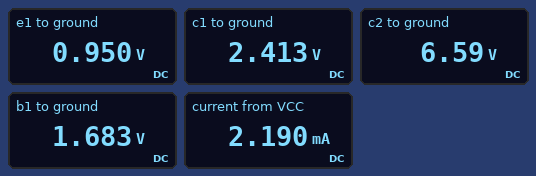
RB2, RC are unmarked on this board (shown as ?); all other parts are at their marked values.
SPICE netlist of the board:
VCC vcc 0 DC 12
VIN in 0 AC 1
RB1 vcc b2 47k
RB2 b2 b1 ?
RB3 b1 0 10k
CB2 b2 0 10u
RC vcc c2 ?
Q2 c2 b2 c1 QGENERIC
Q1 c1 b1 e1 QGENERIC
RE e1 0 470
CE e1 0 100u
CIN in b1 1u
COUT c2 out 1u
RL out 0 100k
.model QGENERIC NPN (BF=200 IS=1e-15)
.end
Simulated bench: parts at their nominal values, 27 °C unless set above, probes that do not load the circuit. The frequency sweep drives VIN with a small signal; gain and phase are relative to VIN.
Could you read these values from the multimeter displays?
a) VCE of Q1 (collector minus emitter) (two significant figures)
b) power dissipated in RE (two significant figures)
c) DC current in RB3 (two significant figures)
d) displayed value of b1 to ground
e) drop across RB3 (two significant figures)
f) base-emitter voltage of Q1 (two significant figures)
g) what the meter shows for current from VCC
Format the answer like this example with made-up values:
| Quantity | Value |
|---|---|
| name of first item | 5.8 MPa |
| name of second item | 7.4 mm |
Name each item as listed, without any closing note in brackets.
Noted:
| Quantity | Value |
|---|---|
| VCE of Q1 (collector minus emitter) | 1.5 V |
| power dissipated in RE | 1.9 mW |
| DC current in RB3 | 170 µA |
| displayed value of b1 to ground | 1.683 V |
| drop across RB3 | 1.7 V |
| base-emitter voltage of Q1 | 730 mV |
| what the meter shows for current from VCC | 2.190 mA |
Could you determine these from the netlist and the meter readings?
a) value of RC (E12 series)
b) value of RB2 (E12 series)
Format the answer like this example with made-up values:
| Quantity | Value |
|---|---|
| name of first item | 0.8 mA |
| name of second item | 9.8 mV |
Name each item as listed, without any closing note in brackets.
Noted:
| Quantity | Value |
|---|---|
| value of RC | 2.7 kΩ |
| value of RB2 | 8.2 kΩ |
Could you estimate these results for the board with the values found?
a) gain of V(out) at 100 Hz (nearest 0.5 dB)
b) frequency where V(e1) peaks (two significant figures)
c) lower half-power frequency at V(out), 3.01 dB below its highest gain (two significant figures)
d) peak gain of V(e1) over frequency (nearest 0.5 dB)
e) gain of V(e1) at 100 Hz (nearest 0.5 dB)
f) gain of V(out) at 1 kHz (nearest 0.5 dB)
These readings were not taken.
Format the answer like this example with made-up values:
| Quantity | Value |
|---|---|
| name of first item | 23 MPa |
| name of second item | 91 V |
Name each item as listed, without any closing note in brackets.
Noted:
| Quantity | Value |
|---|---|
| gain of V(out) at 100 Hz | 39.0 dB |
| frequency where V(e1) peaks | 71 Hz |
| lower half-power frequency at V(out), 3.01 dB below its highest gain | 200 Hz |
| peak gain of V(e1) over frequency | -5.0 dB |
| gain of V(e1) at 100 Hz | -5.5 dB |
| gain of V(out) at 1 kHz | 46.0 dB |
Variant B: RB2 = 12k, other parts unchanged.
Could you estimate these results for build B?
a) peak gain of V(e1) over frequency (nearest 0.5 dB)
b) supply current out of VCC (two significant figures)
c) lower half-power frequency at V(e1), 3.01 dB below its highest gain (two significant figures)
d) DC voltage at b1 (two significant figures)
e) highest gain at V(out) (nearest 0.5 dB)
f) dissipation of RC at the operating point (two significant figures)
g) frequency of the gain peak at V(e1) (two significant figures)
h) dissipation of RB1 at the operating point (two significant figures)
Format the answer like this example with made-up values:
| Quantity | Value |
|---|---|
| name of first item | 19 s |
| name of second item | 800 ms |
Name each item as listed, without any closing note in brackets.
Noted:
| Quantity | Value |
|---|---|
| peak gain of V(e1) over frequency | -5.0 dB |
| supply current out of VCC | 2.0 mA |
| lower half-power frequency at V(e1), 3.01 dB below its highest gain | 17 Hz |
| DC voltage at b1 | 1.6 V |
| highest gain at V(out) | 45.5 dB |
| dissipation of RC at the operating point | 9.0 mW |
| frequency of the gain peak at V(e1) | 61 Hz |
| dissipation of RB1 at the operating point | 1.5 mW |
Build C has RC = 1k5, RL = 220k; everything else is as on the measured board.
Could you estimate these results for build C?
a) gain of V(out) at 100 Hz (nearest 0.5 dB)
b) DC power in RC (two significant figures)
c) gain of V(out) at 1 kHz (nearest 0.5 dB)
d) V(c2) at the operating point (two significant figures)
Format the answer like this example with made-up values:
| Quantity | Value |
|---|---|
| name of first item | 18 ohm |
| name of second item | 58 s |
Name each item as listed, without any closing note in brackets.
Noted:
| Quantity | Value |
|---|---|
| gain of V(out) at 100 Hz | 34.0 dB |
| DC power in RC | 6.0 mW |
| gain of V(out) at 1 kHz | 41.0 dB |
| V(c2) at the operating point | 9.0 V |
